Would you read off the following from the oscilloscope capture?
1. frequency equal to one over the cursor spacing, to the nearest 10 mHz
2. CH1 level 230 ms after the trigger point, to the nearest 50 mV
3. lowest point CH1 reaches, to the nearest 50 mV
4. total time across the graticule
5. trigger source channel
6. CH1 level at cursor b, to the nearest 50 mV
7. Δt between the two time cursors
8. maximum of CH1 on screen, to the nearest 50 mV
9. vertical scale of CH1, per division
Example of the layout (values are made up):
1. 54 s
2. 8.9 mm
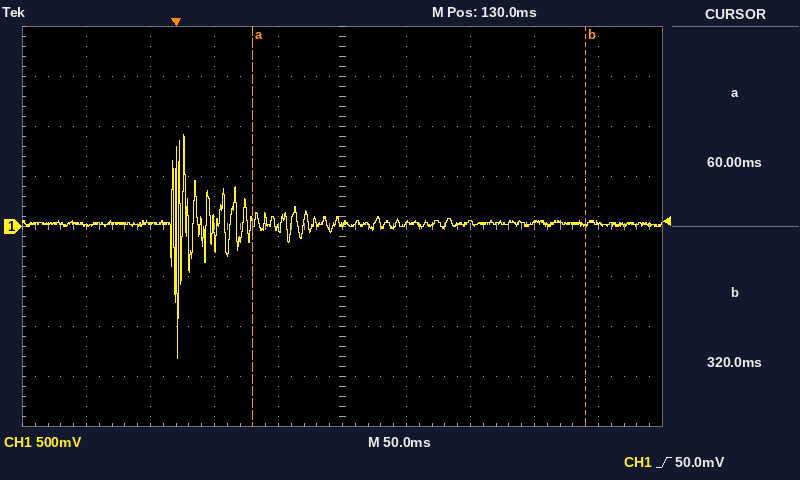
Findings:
1. 3.85 Hz
2. 50 mV
3. -1.30 V
4. 500 ms
5. CH1
6. 0 mV
7. 260 ms
8. 900 mV
9. 500 mV
